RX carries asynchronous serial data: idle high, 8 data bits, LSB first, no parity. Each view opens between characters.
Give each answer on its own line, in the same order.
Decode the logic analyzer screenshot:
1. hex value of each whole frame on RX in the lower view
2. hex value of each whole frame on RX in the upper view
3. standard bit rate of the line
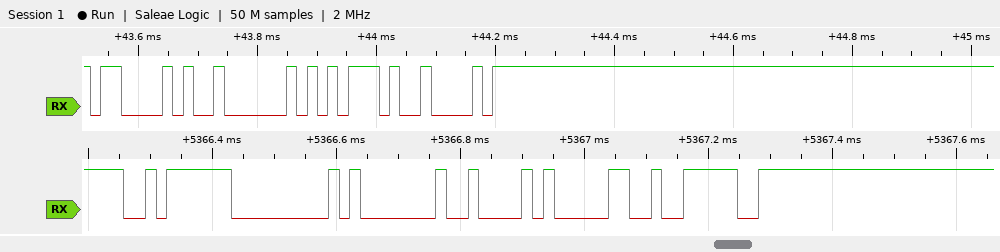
FA, 00, 01, 42, 30, 3E
43, 02, 75, 42
57600 baud
